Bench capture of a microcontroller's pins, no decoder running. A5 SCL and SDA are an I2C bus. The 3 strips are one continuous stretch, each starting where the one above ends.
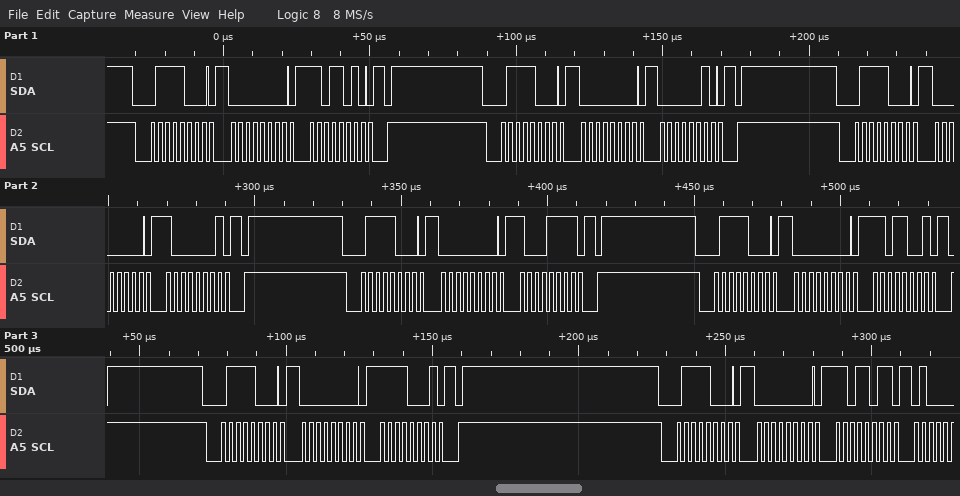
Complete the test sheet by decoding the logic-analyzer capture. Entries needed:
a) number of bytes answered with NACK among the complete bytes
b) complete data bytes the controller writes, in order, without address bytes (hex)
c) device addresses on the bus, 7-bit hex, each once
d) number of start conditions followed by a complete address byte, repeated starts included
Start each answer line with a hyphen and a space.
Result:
- 0
- 00 DA 00 02 00 81 00 8F 00 D9 00 F1 00 DB
- 0x3C
- 7
